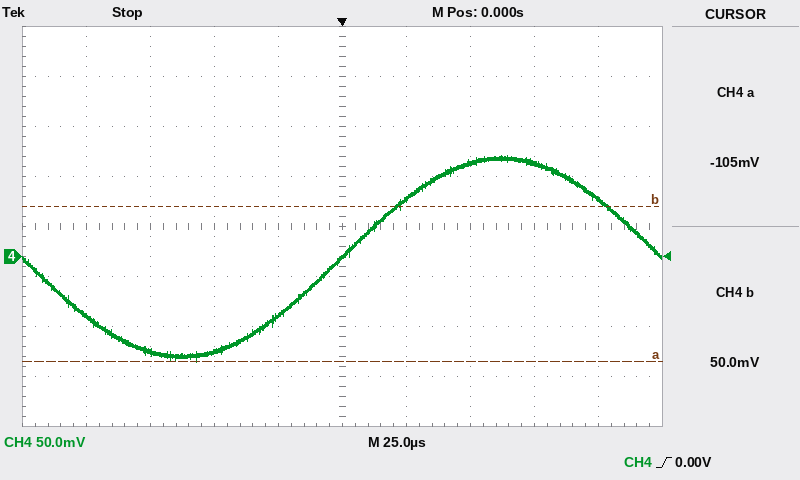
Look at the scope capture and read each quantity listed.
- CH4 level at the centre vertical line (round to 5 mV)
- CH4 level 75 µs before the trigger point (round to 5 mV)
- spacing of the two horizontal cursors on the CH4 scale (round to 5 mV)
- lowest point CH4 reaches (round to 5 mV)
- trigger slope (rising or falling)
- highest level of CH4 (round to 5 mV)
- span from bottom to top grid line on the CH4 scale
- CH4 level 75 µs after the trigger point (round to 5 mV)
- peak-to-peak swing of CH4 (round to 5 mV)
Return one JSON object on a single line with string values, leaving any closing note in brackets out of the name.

{"CH4 level at the centre vertical line": "0 mV", "CH4 level 75 µs before the trigger point": "-95 mV", "spacing of the two horizontal cursors on the CH4 scale": "155 mV", "lowest point CH4 reaches": "-105 mV", "trigger slope": "rising", "highest level of CH4": "100 mV", "span from bottom to top grid line on the CH4 scale": "400 mV", "CH4 level 75 µs after the trigger point": "95 mV", "peak-to-peak swing of CH4": "205 mV"}
